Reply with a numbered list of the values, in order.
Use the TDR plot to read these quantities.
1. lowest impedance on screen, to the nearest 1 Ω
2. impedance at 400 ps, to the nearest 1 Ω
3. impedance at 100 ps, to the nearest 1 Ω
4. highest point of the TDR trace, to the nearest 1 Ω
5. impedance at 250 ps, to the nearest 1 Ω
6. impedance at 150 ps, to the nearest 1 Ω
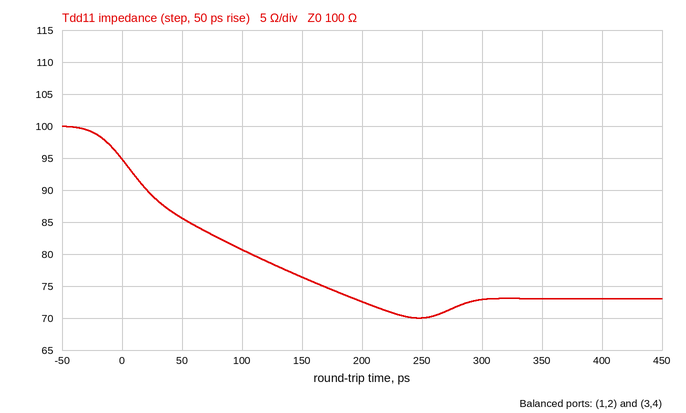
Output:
1. 70 Ω
2. 73 Ω
3. 81 Ω
4. 100 Ω
5. 70 Ω
6. 76 Ω
